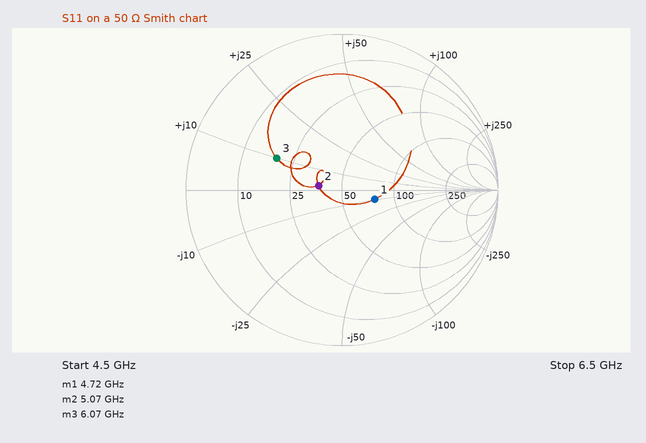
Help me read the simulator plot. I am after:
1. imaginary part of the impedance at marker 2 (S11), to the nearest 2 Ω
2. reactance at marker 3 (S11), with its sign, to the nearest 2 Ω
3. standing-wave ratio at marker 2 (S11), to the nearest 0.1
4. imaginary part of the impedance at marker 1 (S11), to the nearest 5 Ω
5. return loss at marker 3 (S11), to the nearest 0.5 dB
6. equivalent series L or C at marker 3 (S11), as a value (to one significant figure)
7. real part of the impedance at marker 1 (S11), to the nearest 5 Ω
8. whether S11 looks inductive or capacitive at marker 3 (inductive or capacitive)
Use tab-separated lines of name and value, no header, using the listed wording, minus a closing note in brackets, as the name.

imaginary part of the impedance at marker 2 (S11), to the nearest 2 Ω	+2 Ω
reactance at marker 3 (S11), with its sign, to the nearest 2 Ω	+10 Ω
standing-wave ratio at marker 2 (S11), to the nearest 0.1	1.4
imaginary part of the impedance at marker 1 (S11), to the nearest 5 Ω	-10 Ω
return loss at marker 3 (S11), to the nearest 0.5 dB	6.5 dB
equivalent series L or C at marker 3 (S11), as a value	300 pH
real part of the impedance at marker 1 (S11), to the nearest 5 Ω	75 Ω
whether S11 looks inductive or capacitive at marker 3	inductive
